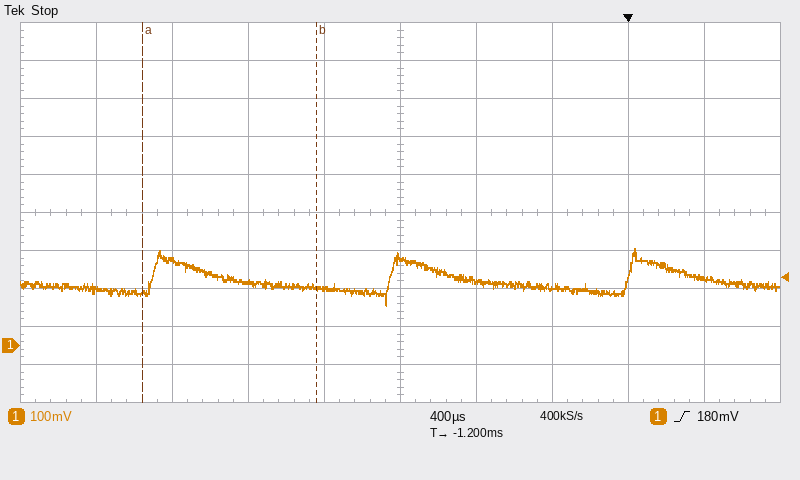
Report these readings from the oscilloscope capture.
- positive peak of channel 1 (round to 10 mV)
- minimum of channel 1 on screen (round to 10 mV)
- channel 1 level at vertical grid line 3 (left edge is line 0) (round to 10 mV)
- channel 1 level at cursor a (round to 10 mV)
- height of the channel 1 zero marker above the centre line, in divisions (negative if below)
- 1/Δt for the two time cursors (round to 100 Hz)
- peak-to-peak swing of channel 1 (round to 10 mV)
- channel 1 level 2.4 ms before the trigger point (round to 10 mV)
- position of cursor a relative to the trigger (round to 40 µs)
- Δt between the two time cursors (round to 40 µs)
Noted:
260 mV
110 mV
170 mV
140 mV
-3.5 div
1.1 kHz
150 mV
220 mV
-2.56 ms
920 µs
